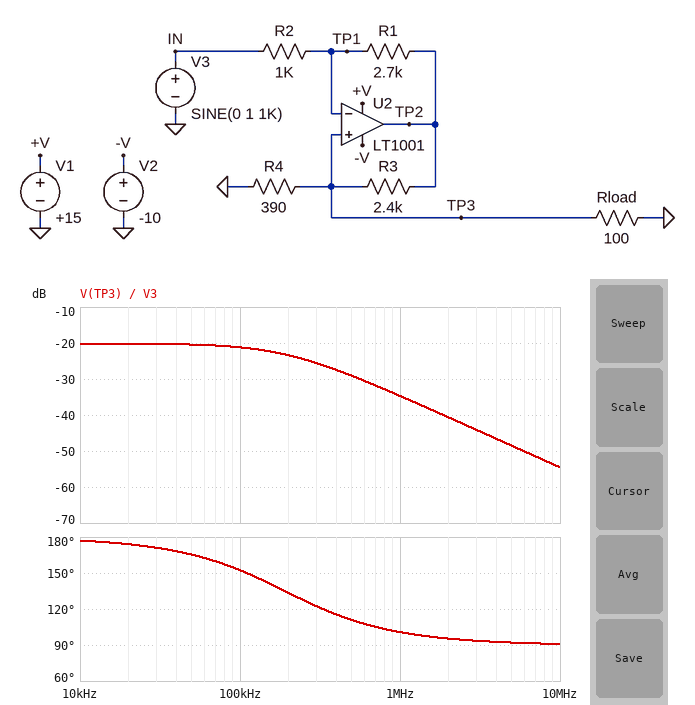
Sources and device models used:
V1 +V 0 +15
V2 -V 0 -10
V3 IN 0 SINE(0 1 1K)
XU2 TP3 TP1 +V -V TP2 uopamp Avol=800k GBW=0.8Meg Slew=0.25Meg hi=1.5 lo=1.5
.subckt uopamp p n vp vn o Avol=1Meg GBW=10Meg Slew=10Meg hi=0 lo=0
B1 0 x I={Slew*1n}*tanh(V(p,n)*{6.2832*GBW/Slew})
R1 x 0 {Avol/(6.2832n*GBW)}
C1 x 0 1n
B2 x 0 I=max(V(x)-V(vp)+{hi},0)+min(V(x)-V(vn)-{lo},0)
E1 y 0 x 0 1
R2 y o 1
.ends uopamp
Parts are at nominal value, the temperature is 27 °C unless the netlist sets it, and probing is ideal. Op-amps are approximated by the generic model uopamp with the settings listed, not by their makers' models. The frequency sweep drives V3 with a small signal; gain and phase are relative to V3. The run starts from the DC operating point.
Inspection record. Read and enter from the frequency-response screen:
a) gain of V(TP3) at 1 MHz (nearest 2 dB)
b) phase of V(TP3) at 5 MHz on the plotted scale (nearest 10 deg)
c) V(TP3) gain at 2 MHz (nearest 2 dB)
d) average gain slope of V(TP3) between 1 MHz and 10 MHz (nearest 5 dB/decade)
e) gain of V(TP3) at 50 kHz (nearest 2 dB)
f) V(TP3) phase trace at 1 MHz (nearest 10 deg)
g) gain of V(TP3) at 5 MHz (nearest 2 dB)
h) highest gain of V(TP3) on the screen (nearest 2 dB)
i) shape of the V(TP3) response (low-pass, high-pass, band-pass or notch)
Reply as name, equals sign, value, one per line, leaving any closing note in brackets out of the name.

gain of V(TP3) at 1 MHz = -34 dB
phase of V(TP3) at 5 MHz on the plotted scale = 90 deg
V(TP3) gain at 2 MHz = -40 dB
average gain slope of V(TP3) between 1 MHz and 10 MHz = -20 dB/decade
gain of V(TP3) at 50 kHz = -20 dB
V(TP3) phase trace at 1 MHz = 100 deg
gain of V(TP3) at 5 MHz = -48 dB
highest gain of V(TP3) on the screen = -20 dB
shape of the V(TP3) response = low-pass
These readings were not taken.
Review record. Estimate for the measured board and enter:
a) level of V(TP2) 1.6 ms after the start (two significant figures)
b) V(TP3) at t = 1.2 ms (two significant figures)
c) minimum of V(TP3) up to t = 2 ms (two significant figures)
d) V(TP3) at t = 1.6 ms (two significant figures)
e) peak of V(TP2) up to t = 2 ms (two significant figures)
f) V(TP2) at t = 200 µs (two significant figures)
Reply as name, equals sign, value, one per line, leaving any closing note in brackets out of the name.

level of V(TP2) 1.6 ms after the start = 1.8 V
V(TP3) at t = 1.2 ms = -93 mV
minimum of V(TP3) up to t = 2 ms = -98 mV
V(TP3) at t = 1.6 ms = 57 mV
peak of V(TP2) up to t = 2 ms = 3.1 V
V(TP2) at t = 200 µs = -2.9 V
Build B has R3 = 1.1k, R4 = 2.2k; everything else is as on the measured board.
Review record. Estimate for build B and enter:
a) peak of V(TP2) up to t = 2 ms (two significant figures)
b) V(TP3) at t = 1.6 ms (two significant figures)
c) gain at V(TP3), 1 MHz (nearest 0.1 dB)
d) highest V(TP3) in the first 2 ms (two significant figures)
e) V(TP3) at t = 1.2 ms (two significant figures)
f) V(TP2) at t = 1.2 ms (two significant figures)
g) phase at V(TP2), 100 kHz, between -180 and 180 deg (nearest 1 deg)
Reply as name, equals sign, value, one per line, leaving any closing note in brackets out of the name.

peak of V(TP2) up to t = 2 ms = 3.8 V
V(TP3) at t = 1.6 ms = 180 mV
gain at V(TP3), 1 MHz = -26.7 dB
highest V(TP3) in the first 2 ms = 310 mV
V(TP3) at t = 1.2 ms = -290 mV
V(TP2) at t = 1.2 ms = -3.6 V
phase at V(TP2), 100 kHz, between -180 and 180 deg = 147 deg
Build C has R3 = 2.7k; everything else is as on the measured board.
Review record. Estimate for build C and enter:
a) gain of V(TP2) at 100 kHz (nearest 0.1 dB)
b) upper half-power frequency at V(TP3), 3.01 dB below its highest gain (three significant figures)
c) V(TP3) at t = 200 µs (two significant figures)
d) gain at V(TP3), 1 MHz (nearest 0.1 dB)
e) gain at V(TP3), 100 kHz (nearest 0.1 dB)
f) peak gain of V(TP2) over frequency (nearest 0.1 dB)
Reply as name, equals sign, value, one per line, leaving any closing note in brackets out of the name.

gain of V(TP2) at 100 kHz = 8.6 dB
upper half-power frequency at V(TP3), 3.01 dB below its highest gain = 193 kHz
V(TP3) at t = 200 µs = -82 mV
gain at V(TP3), 1 MHz = -35.7 dB
gain at V(TP3), 100 kHz = -22.3 dB
peak gain of V(TP2) over frequency = 9.6 dB
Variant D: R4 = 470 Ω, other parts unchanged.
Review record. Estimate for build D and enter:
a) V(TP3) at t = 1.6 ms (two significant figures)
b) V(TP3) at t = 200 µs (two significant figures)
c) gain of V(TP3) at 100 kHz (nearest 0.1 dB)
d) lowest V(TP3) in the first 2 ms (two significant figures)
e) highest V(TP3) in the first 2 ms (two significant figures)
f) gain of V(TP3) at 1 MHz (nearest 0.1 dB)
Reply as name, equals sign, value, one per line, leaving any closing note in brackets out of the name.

V(TP3) at t = 1.6 ms = 60 mV
V(TP3) at t = 200 µs = -97 mV
gain of V(TP3) at 100 kHz = -20.9 dB
lowest V(TP3) in the first 2 ms = -100 mV
highest V(TP3) in the first 2 ms = 100 mV
gain of V(TP3) at 1 MHz = -34.4 dB
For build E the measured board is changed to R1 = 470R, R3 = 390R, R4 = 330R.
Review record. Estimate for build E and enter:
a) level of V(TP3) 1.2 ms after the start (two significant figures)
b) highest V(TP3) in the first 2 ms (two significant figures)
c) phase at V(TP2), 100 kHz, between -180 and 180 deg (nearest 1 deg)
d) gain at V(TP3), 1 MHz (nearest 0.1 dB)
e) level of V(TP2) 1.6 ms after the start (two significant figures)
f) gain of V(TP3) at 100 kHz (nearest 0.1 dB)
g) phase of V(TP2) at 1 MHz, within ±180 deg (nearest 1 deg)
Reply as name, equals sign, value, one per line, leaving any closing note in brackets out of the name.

level of V(TP3) 1.2 ms after the start = -97 mV
highest V(TP3) in the first 2 ms = 100 mV
phase at V(TP2), 100 kHz, between -180 and 180 deg = 166 deg
gain at V(TP3), 1 MHz = -28.2 dB
level of V(TP2) 1.6 ms after the start = 360 mV
gain of V(TP3) at 100 kHz = -20.1 dB
phase of V(TP2) at 1 MHz, within ±180 deg = 112 deg
